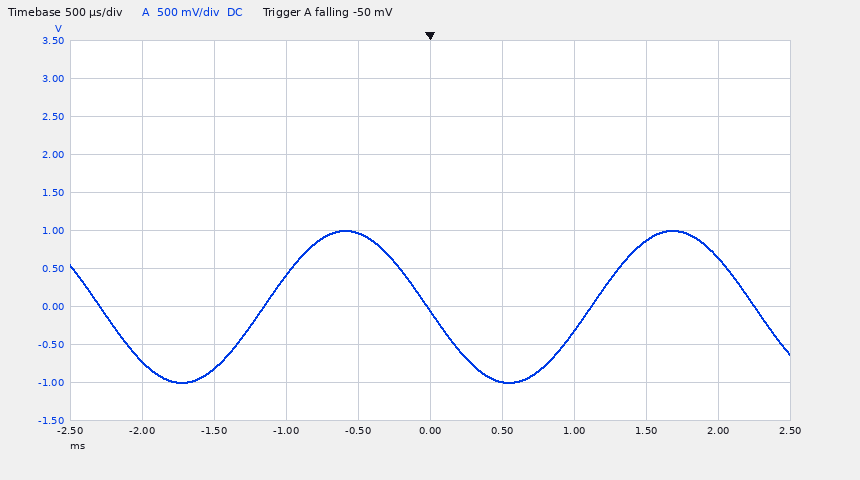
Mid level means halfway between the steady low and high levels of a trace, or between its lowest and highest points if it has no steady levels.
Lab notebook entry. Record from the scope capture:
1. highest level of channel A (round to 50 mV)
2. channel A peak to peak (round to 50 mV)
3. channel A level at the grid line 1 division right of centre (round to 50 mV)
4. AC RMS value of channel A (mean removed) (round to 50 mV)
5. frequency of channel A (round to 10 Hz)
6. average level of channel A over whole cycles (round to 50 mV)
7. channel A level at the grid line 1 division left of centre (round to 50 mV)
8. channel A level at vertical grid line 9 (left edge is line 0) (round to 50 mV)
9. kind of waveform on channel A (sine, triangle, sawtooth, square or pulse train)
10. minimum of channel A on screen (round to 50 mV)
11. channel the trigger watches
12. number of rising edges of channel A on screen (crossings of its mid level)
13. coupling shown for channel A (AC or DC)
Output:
1.00 V
2.00 V
-1.00 V
700 mV
440 Hz
0 mV
950 mV
650 mV
sine
-1.00 V
channel A
2
DC
